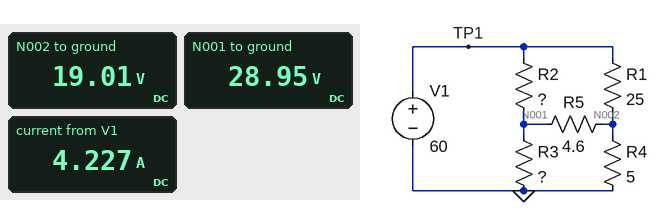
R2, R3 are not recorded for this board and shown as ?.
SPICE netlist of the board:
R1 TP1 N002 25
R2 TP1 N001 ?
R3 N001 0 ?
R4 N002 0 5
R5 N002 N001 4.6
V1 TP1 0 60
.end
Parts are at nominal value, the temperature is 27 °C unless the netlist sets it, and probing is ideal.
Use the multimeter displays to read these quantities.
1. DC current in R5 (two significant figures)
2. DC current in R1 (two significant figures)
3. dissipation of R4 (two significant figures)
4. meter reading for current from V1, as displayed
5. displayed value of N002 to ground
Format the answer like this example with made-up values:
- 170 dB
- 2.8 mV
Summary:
- 2.2 A
- 1.6 A
- 72 W
- 4.227 A
- 19.01 V
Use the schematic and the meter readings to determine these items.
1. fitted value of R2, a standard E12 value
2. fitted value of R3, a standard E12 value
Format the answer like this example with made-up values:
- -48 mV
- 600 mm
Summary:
- 12 Ω
- 68 Ω
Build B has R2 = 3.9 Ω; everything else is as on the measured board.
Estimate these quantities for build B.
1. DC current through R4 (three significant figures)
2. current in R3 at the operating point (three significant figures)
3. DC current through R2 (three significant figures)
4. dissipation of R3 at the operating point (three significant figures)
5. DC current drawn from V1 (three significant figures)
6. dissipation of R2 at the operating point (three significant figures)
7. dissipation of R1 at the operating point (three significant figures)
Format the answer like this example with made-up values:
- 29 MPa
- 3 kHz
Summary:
- 5.13 A
- 631 mA
- 4.38 A
- 27.1 W
- 5.76 A
- 75.0 W
- 47.2 W
